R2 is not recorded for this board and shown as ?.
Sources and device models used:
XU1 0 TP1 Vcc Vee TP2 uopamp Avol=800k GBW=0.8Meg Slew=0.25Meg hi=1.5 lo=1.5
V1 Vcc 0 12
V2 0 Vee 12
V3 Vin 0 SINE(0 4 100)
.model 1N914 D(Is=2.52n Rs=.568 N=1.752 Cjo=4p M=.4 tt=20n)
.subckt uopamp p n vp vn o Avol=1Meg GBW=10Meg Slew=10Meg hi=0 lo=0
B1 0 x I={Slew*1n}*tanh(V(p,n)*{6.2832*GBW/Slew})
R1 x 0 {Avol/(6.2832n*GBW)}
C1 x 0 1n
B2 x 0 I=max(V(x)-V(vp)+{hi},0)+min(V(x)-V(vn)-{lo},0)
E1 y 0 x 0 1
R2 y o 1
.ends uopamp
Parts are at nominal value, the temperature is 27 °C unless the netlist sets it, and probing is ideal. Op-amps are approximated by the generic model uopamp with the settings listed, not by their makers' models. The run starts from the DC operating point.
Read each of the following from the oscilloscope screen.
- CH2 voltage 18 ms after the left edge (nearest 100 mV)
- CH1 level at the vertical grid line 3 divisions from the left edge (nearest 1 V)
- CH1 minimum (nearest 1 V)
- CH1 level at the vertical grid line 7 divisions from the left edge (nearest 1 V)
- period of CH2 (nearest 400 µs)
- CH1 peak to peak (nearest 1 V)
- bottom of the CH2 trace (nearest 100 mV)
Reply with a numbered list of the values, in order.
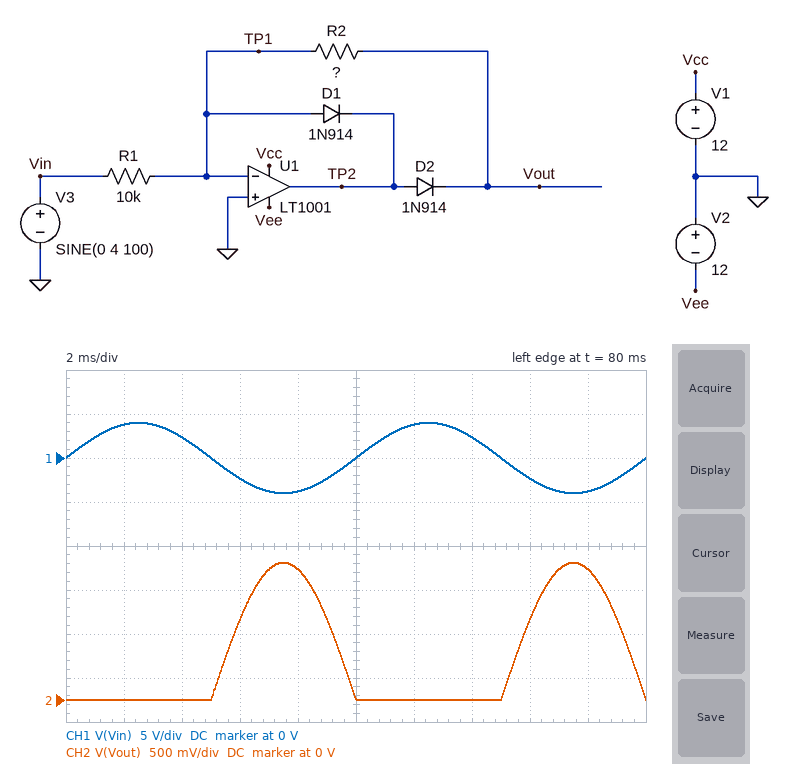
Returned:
1. 1.5 V
2. -2 V
3. -4 V
4. 2 V
5. 10.0 ms
6. 8 V
7. 0 V
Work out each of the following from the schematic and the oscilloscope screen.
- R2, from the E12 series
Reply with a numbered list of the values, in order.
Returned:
1. 3.9 kΩ
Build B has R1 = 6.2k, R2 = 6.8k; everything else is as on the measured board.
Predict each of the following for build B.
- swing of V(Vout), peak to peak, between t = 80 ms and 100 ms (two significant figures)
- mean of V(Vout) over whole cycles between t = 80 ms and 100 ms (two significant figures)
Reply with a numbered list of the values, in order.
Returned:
1. 4.4 V
2. 1.4 V
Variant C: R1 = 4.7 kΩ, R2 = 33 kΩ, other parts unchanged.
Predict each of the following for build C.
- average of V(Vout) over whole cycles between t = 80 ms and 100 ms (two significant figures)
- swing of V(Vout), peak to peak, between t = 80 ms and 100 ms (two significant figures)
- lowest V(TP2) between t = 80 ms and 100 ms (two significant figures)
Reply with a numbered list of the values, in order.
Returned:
1. 4.4 V
2. 10 V
3. -580 mV
